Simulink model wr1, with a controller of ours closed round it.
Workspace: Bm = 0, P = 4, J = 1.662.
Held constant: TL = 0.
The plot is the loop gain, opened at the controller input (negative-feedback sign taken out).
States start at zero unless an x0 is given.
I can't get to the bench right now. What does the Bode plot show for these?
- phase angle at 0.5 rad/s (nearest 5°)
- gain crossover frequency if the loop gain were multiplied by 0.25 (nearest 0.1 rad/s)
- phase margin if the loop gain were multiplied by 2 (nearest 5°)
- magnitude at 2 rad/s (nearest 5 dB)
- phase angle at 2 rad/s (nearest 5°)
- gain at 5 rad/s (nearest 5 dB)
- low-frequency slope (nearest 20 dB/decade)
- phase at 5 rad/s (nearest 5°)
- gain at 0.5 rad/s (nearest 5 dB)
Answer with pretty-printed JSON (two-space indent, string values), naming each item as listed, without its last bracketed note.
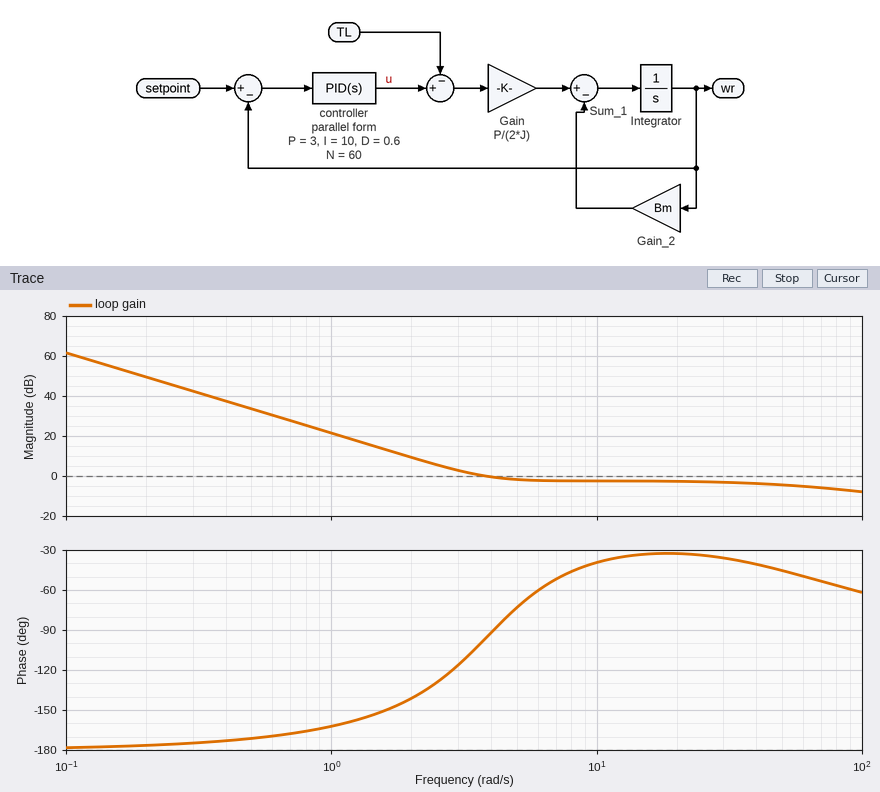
{
  "phase angle at 0.5 rad/s": "-170°",
  "gain crossover frequency if the loop gain were multiplied by 0.25": "1.7 rad/s",
  "phase margin if the loop gain were multiplied by 2": "125°",
  "magnitude at 2 rad/s": "10 dB",
  "phase angle at 2 rad/s": "-140°",
  "gain at 5 rad/s": "0 dB",
  "low-frequency slope": "-40 dB/decade",
  "phase at 5 rad/s": "-75°",
  "gain at 0.5 rad/s": "35 dB"
}
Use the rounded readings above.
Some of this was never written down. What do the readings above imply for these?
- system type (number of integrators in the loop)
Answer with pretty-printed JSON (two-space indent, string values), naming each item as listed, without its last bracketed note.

{
  "system type": "2"
}
